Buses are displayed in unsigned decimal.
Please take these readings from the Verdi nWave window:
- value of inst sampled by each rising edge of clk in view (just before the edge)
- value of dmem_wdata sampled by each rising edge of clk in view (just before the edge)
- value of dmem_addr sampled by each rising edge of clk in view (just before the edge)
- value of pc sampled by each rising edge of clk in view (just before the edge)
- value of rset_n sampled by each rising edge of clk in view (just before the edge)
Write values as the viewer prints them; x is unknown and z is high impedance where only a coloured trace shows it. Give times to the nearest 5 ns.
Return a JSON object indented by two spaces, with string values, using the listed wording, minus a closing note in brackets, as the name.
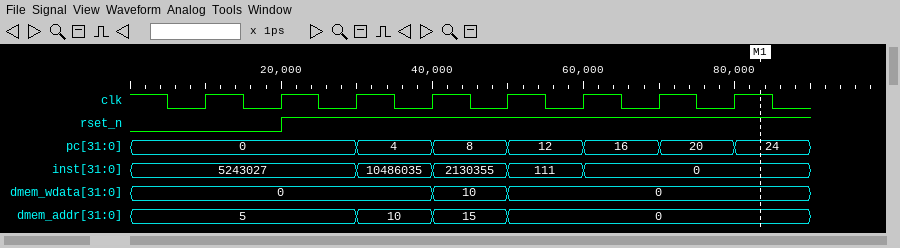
{
  "value of inst sampled by each rising edge of clk in view": "5243027, 5243027, 5243027, 10486035, 2130355, 111, 0, 0",
  "value of dmem_wdata sampled by each rising edge of clk in view": "0, 0, 0, 0, 10, 0, 0, 0",
  "value of dmem_addr sampled by each rising edge of clk in view": "5, 5, 5, 10, 15, 0, 0, 0",
  "value of pc sampled by each rising edge of clk in view": "0, 0, 0, 4, 8, 12, 16, 20",
  "value of rset_n sampled by each rising edge of clk in view": "0 0 1 1 1 1 1 1"
}
